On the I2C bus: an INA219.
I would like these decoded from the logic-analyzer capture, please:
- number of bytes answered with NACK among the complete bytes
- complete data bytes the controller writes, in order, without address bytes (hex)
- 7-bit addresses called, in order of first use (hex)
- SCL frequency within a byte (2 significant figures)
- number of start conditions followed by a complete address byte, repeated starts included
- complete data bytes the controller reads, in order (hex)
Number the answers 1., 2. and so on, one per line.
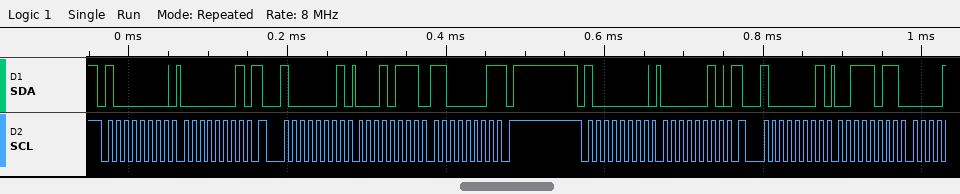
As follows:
1. 1
2. 01 02
3. 0x40
4. 100 kHz
5. 4
6. 17 C1 3B
